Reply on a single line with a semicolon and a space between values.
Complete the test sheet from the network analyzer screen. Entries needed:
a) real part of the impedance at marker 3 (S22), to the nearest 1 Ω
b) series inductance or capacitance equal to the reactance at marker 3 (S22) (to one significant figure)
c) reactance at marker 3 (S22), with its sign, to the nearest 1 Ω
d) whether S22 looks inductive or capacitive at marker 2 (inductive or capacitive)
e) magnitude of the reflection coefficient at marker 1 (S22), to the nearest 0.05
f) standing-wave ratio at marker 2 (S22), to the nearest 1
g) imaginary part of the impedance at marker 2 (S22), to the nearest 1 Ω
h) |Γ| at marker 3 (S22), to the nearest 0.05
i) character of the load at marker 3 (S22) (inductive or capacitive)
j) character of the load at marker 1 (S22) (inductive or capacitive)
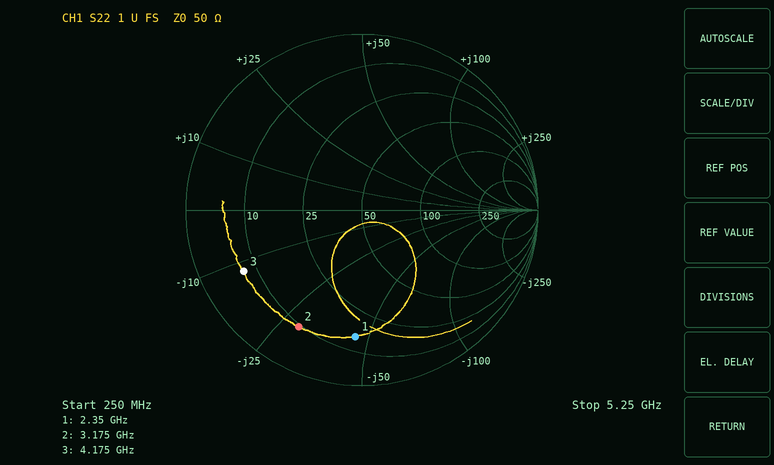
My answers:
7 Ω; 3 pF; -12 Ω; capacitive; 0.70; 7; -29 Ω; 0.75; capacitive; capacitive
